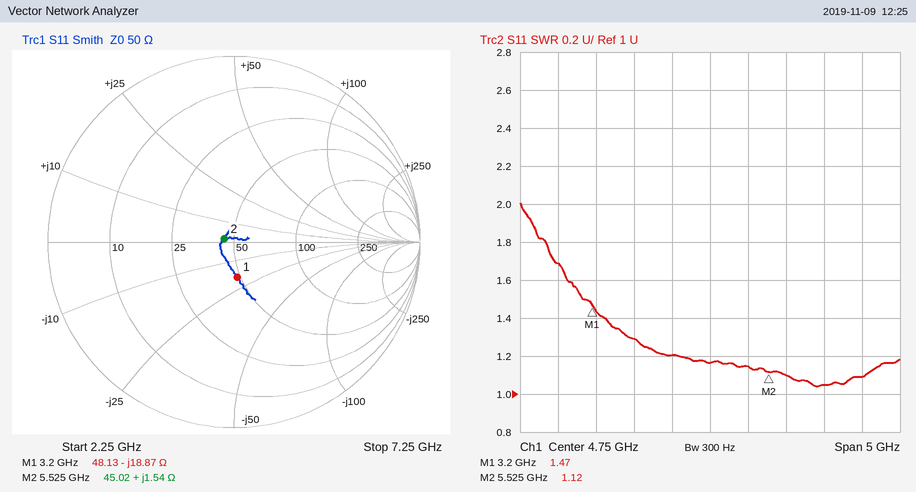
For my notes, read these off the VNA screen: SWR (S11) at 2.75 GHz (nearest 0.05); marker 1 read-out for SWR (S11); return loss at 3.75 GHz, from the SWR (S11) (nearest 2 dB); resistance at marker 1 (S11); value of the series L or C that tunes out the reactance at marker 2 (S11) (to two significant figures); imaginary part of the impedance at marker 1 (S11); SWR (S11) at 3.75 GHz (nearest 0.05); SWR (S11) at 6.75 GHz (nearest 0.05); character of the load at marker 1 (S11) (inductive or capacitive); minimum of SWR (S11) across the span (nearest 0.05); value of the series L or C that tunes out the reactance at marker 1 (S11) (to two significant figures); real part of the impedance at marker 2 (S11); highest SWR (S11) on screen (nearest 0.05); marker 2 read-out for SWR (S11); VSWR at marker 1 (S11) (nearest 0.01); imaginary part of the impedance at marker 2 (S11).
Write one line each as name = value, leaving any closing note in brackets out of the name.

SWR (S11) at 2.75 GHz = 1.70
marker 1 read-out for SWR = 1.47
return loss at 3.75 GHz, from the SWR (S11) = 18 dB
resistance at marker 1 = 48.13 Ω
value of the series L or C that tunes out the reactance at marker 2 (S11) = 19 pF
imaginary part of the impedance at marker 1 = -18.87 Ω
SWR (S11) at 3.75 GHz = 1.30
SWR (S11) at 6.75 GHz = 1.10
character of the load at marker 1 (S11) = capacitive
minimum of SWR (S11) across the span = 1.05
value of the series L or C that tunes out the reactance at marker 1 (S11) = 940 pH
real part of the impedance at marker 2 = 45.02 Ω
highest SWR (S11) on screen = 2.00
marker 2 read-out for SWR = 1.12
VSWR at marker 1 (S11) = 1.47
imaginary part of the impedance at marker 2 = +1.54 Ω
